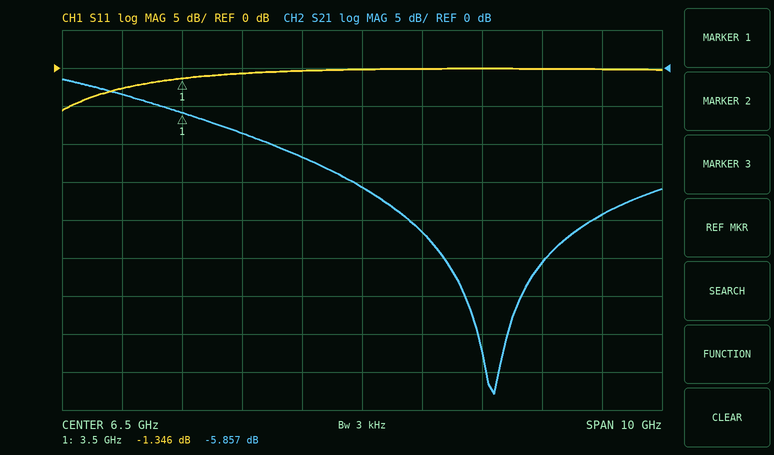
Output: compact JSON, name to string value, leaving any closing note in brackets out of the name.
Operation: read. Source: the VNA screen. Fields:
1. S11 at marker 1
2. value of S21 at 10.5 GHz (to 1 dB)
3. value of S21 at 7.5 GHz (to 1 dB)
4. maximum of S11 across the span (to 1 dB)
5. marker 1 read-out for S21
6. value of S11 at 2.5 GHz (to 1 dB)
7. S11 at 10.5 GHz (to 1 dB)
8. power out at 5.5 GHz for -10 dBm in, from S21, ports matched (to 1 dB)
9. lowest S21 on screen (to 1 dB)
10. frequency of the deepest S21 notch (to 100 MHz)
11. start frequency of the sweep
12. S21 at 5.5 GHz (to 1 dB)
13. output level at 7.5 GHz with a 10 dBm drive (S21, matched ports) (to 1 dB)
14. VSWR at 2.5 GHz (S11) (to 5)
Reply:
{"S11 at marker 1": "-1.346 dB", "value of S21 at 10.5 GHz": "-19 dB", "value of S21 at 7.5 GHz": "-22 dB", "maximum of S11 across the span": "0 dB", "marker 1 read-out for S21": "-5.857 dB", "value of S11 at 2.5 GHz": "-3 dB", "S11 at 10.5 GHz": "0 dB", "power out at 5.5 GHz for -10 dBm in, from S21, ports matched": "-22 dBm", "lowest S21 on screen": "-43 dB", "frequency of the deepest S21 notch": "8.7 GHz", "start frequency of the sweep": "1.5 GHz", "S21 at 5.5 GHz": "-12 dB", "output level at 7.5 GHz with a 10 dBm drive (S21, matched ports)": "-12 dBm", "VSWR at 2.5 GHz (S11)": "5"}
